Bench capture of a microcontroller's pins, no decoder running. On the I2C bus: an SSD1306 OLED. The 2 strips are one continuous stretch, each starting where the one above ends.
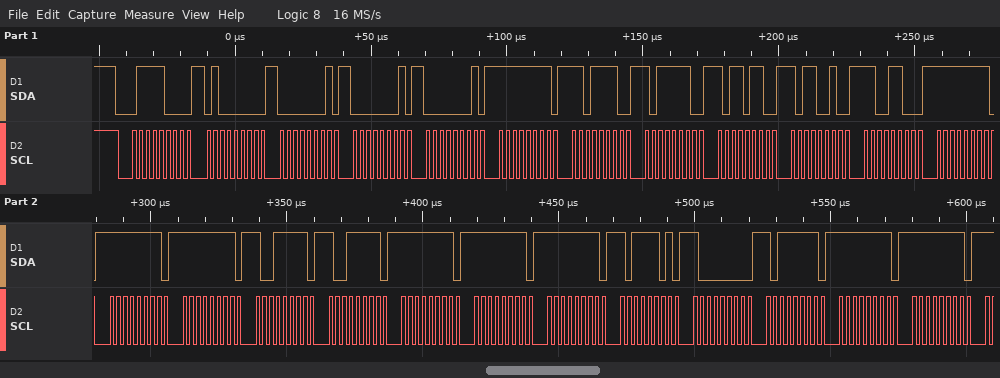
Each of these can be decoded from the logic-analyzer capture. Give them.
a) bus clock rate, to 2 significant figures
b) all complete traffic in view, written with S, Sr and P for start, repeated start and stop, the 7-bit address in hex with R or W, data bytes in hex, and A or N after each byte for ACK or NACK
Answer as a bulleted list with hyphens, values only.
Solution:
- 400 kHz
- S 3CW A 40 A 01 A 01 A 01 A FF A DE A BE A B6 A B2 A CC A FF A FF A FF A 9F A 9F A FF A FF A FF A BD A 80 A BF A FF A FF A
